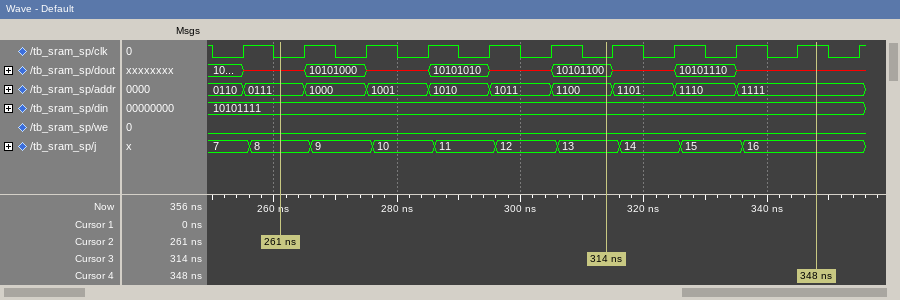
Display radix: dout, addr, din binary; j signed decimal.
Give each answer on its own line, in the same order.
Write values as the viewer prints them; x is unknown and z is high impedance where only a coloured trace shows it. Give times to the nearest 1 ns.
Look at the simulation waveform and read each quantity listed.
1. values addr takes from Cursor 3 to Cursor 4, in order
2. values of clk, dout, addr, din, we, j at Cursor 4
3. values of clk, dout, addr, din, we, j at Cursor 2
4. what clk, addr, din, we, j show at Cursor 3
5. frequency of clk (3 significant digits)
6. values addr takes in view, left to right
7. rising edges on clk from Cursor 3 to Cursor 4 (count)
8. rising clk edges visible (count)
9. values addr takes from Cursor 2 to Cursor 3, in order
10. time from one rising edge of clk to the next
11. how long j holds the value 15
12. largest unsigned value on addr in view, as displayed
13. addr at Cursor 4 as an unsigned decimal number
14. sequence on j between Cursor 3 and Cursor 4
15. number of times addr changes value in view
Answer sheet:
1100, 1101, 1110, 1111
clk=1, dout=x, addr=1111, din=10101111, we=0, j=16
clk=0, dout=x, addr=0111, din=10101111, we=0, j=8
clk=0, addr=1100, din=10101111, we=0, j=13
100 MHz
0110, 0111, 1000, 1001, 1010, 1011, 1100, 1101, 1110, 1111
4
11
0111, 1000, 1001, 1010, 1011, 1100
10 ns
10 ns
1111
15
13, 14, 15, 16
9
